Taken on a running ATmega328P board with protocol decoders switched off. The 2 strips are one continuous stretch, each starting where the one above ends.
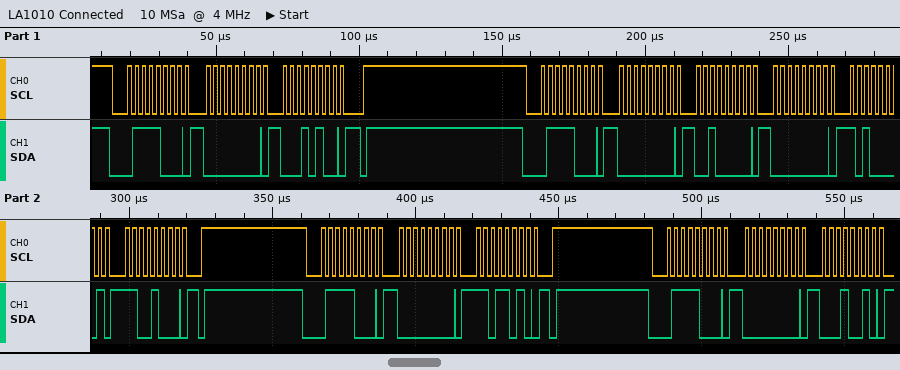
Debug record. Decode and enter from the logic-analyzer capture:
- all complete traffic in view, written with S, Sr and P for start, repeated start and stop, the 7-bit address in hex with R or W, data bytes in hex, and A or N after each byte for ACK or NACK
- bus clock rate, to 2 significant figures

S 3CW A 00 A 14 A P S 3CW A 00 A 20 A 00 A A1 A C8 A P S 3CW A 00 A DA A P S 3CW A 00 A 12 A
400 kHz
